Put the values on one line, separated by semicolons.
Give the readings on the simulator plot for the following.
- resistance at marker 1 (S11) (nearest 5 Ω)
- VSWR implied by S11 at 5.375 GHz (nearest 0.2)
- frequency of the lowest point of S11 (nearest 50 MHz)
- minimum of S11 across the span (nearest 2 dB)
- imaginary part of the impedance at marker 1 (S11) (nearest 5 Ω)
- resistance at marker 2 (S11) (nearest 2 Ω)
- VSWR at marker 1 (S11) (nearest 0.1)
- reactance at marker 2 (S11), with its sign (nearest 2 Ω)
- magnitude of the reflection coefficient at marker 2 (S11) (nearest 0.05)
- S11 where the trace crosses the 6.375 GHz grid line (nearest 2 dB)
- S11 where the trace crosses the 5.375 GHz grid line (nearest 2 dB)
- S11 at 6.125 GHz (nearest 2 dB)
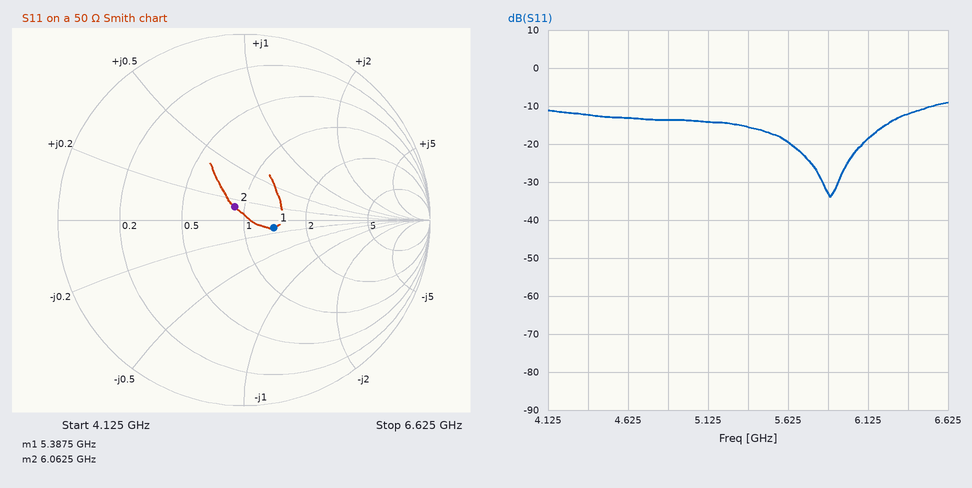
70 Ω; 1.4; 5.90 GHz; -34 dB; -5 Ω; 44 Ω; 1.4; +6 Ω; 0.10; -12 dB; -16 dB; -18 dB
